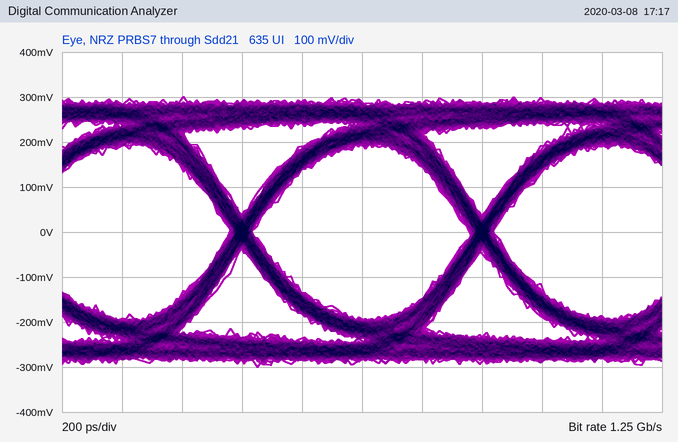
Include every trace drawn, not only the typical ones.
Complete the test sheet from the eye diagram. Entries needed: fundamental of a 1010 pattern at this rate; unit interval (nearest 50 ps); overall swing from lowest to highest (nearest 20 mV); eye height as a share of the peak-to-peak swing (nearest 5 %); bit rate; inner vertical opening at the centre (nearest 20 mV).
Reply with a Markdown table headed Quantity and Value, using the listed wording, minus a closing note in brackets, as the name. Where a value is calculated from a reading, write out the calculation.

| Quantity | Value |
|---|---|
| fundamental of a 1010 pattern at this rate | 625 MHz |
| unit interval | 800 ps |
| overall swing from lowest to highest | 600 mV |
| eye height as a share of the peak-to-peak swing | 380 mV / 600 mV ≈ 63.3 %, so 65 % to the nearest 5 % |
| bit rate | 1.25 Gb/s |
| inner vertical opening at the centre | 380 mV |
